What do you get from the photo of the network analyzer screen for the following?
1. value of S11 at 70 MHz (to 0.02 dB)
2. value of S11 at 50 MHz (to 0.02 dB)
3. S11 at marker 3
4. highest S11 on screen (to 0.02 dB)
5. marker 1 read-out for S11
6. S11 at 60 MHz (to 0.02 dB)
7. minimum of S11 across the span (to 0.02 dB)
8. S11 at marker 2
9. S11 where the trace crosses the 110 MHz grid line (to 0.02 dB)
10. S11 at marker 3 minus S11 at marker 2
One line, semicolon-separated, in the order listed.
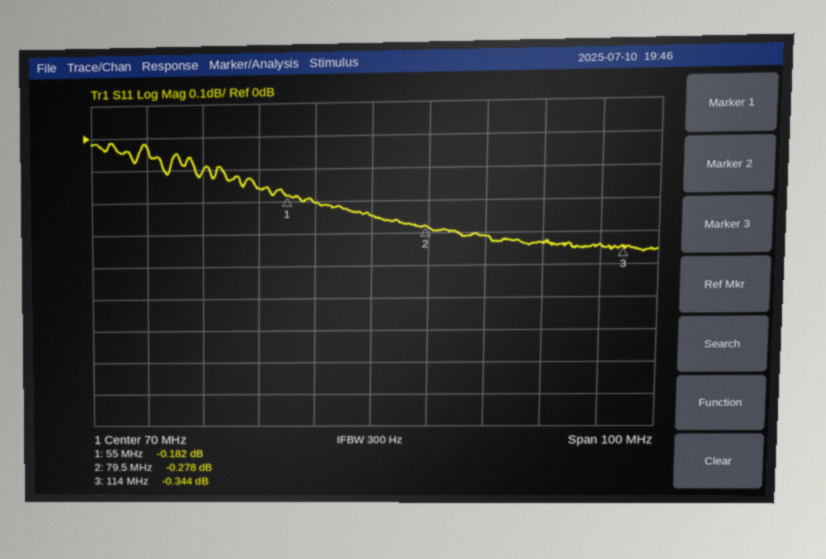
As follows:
-0.24 dB; -0.16 dB; -0.344 dB; -0.02 dB; -0.182 dB; -0.20 dB; -0.36 dB; -0.278 dB; -0.34 dB; -0.066 dB
